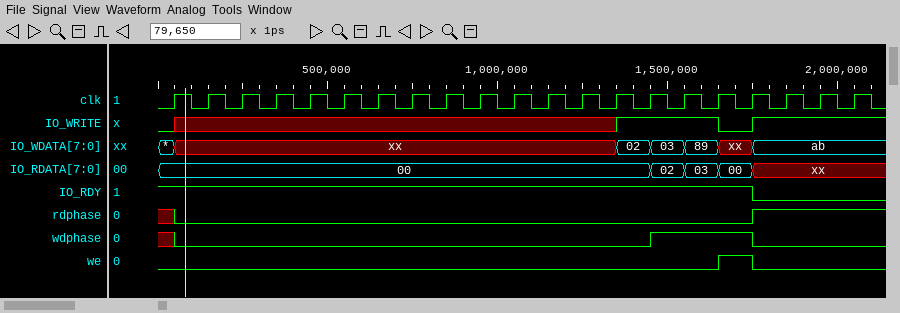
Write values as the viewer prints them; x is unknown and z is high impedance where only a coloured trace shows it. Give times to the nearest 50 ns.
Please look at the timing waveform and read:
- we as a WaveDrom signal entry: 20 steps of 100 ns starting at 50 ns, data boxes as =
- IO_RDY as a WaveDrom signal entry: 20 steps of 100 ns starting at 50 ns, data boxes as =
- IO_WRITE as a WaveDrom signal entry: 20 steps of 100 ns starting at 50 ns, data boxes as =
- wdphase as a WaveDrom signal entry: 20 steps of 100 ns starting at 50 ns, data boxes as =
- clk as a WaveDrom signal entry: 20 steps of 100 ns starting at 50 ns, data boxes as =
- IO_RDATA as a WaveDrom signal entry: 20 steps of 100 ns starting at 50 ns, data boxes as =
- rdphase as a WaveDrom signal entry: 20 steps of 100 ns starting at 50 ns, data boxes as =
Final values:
{name: 'we', wave: '0...............10..'}
{name: 'IO_RDY', wave: '1................0..'}
{name: 'IO_WRITE', wave: 'x............1..01..'}
{name: 'wdphase', wave: '0.............1..0..'}
{name: 'clk', wave: 'p...................'}
{name: 'IO_RDATA', wave: '=.............===x..', data: '00 02 03 00'}
{name: 'rdphase', wave: '0................1..'}
